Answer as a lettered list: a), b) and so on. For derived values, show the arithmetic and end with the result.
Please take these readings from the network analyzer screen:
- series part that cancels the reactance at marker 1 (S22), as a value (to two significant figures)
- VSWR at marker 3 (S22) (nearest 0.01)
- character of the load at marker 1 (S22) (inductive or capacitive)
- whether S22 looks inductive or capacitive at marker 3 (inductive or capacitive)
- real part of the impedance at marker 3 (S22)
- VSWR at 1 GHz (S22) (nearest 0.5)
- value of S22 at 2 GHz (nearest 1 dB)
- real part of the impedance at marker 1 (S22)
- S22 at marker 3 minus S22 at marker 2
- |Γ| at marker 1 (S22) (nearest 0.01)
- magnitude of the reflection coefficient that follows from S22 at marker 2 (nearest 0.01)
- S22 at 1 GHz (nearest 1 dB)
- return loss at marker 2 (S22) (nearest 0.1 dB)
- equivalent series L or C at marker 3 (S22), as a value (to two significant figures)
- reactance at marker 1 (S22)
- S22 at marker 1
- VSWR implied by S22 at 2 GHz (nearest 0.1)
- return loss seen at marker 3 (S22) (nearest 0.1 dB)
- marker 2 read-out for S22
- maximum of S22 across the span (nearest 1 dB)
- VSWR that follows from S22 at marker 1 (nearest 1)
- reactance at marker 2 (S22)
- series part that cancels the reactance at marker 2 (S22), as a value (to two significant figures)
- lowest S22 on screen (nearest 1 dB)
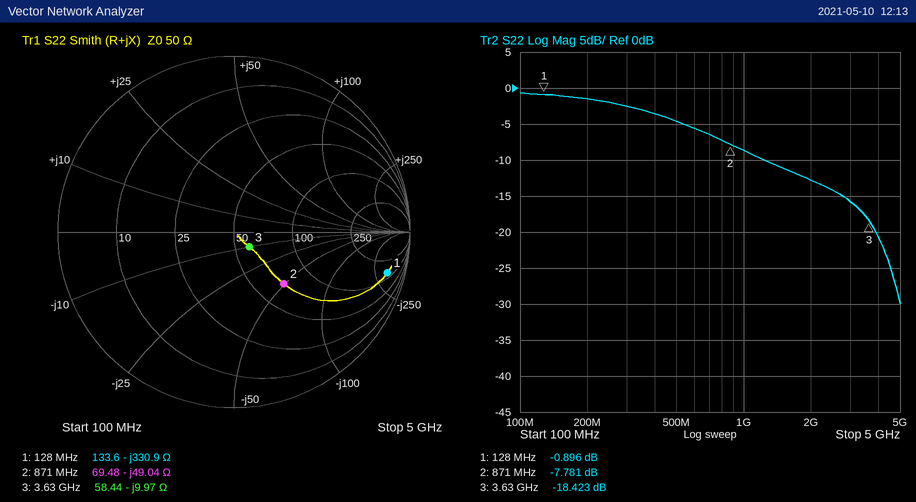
a) L = 330.9 Ω/(2π × 128 MHz) ≈ 411 nH, so 410 nH to two significant figures
b) (1 + 0.1199)/(1 − 0.1199) ≈ 1.27
c) capacitive
d) capacitive
e) 58.44 Ω
f) |Γ| = 10^(-9/20) = 0.3548; VSWR = (1 + 0.3548)/(1 − 0.3548) ≈ 2.10, so 2.0 to the nearest 0.5
g) -13 dB
h) 133.6 Ω
i) -18.423 − (-7.781) = -10.642 dB
j) 0.90
k) 10^(-7.781/20) ≈ 0.41
l) -9 dB
m) 7.8 dB
n) C = 1/(2π × 3.63 GHz × 9.97 Ω) ≈ 4.4 pF
o) -330.9 Ω
p) -0.896 dB
q) |Γ| = 10^(-13/20) = 0.2239; VSWR = (1 + 0.2239)/(1 − 0.2239) ≈ 1.6
r) 18.4 dB
s) -7.781 dB
t) -1 dB
u) (1 + 0.9020)/(1 − 0.9020) ≈ 19
v) -49.04 Ω
w) L = 49.04 Ω/(2π × 871 MHz) ≈ 9.0 nH
x) -30 dB
